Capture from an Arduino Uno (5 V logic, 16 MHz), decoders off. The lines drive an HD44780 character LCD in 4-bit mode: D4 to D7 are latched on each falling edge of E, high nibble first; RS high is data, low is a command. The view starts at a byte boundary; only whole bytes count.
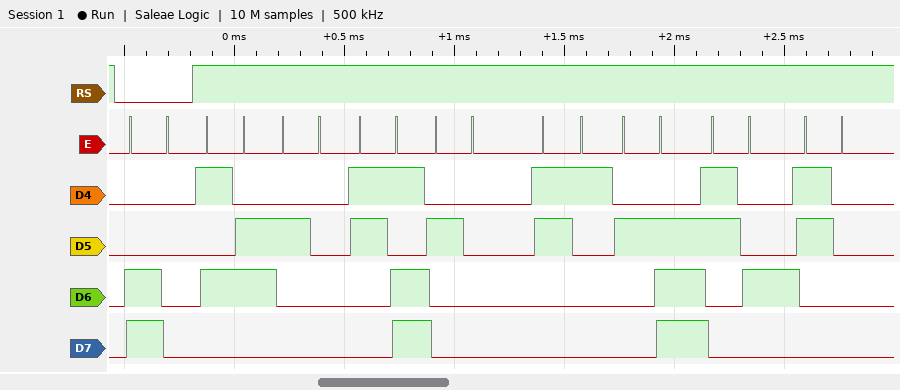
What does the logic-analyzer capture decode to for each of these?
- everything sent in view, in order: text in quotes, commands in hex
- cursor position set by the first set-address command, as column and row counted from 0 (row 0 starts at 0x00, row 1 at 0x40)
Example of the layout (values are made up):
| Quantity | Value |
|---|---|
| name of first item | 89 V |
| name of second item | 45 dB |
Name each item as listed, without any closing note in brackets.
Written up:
| Quantity | Value |
|---|---|
| everything sent in view, in order: text in quotes, commands in hex | 0xC0 "V = 1.40" |
| cursor position set by the first set-address command, as column and row counted from 0 | column 0, row 1 |
